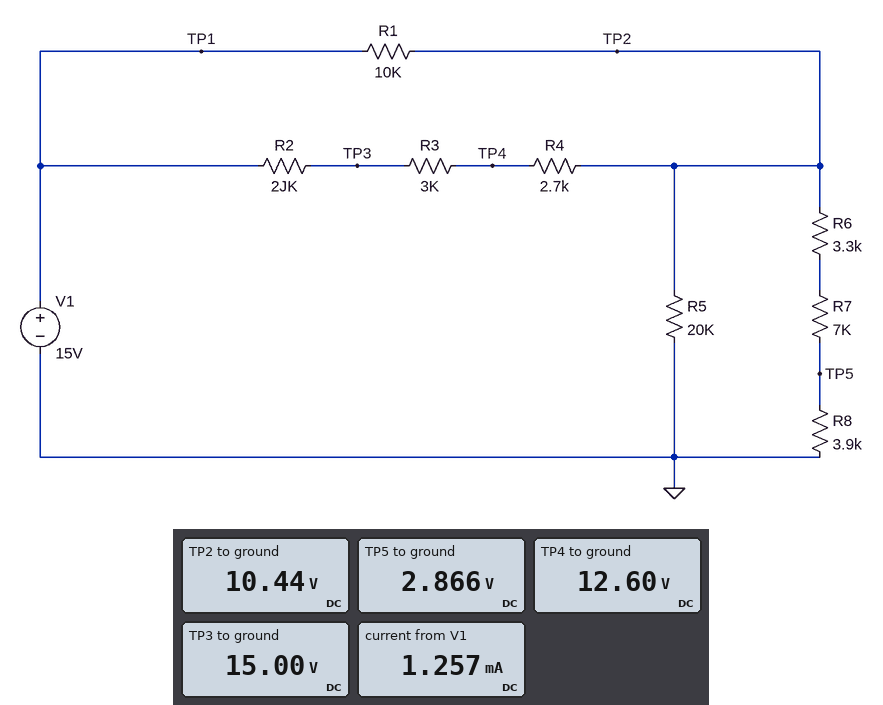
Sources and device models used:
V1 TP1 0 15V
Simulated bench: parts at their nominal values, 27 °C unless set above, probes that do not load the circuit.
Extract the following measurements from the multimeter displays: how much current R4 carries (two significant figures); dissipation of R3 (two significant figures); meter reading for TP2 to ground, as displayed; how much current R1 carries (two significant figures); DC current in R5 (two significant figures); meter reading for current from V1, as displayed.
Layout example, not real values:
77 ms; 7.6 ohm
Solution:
800 µA; 1.9 mW; 10.44 V; 460 µA; 520 µA; 1.257 mA
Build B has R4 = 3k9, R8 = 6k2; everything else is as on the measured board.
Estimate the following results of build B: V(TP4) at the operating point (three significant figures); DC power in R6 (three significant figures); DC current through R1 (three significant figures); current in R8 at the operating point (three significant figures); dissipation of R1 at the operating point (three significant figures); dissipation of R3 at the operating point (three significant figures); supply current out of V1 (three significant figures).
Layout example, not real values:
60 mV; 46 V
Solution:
13.0 V; 1.29 mW; 467 µA; 626 µA; 2.18 mW; 1.37 mW; 1.14 mA
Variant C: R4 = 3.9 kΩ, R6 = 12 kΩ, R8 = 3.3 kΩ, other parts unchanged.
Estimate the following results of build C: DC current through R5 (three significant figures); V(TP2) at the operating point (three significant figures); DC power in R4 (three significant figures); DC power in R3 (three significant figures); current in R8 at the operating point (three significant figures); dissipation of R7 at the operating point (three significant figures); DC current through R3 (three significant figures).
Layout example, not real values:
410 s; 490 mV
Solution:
541 µA; 10.8 V; 1.44 mW; 1.10 mW; 485 µA; 1.65 mW; 607 µA
